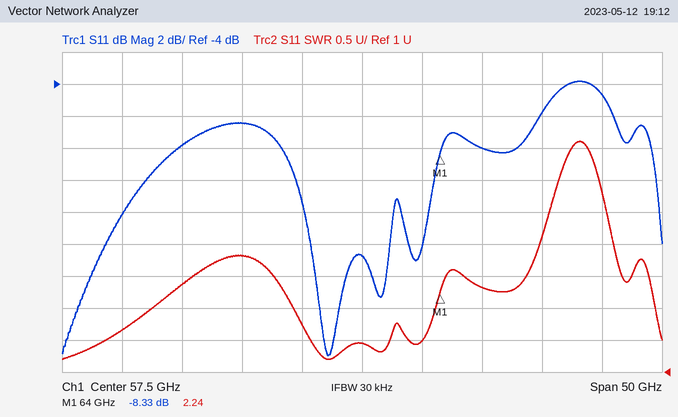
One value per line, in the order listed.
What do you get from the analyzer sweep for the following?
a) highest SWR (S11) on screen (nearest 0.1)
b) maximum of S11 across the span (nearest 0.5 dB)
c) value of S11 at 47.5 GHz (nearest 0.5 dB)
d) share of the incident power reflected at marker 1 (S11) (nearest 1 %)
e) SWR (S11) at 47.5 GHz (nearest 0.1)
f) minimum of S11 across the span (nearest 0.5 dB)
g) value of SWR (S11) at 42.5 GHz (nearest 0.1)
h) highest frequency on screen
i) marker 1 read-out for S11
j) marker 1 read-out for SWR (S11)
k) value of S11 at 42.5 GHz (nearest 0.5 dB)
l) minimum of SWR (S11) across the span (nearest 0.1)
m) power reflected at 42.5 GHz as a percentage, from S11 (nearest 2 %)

4.6
-4.0 dB
-6.5 dB
15 %
2.8
-21.0 dB
2.4
82.5 GHz
-8.33 dB
2.24
-8.0 dB
1.2
16 %
